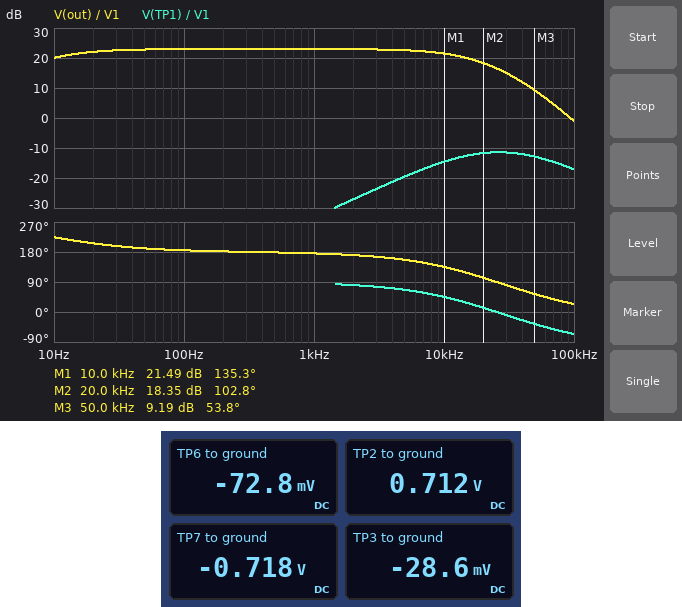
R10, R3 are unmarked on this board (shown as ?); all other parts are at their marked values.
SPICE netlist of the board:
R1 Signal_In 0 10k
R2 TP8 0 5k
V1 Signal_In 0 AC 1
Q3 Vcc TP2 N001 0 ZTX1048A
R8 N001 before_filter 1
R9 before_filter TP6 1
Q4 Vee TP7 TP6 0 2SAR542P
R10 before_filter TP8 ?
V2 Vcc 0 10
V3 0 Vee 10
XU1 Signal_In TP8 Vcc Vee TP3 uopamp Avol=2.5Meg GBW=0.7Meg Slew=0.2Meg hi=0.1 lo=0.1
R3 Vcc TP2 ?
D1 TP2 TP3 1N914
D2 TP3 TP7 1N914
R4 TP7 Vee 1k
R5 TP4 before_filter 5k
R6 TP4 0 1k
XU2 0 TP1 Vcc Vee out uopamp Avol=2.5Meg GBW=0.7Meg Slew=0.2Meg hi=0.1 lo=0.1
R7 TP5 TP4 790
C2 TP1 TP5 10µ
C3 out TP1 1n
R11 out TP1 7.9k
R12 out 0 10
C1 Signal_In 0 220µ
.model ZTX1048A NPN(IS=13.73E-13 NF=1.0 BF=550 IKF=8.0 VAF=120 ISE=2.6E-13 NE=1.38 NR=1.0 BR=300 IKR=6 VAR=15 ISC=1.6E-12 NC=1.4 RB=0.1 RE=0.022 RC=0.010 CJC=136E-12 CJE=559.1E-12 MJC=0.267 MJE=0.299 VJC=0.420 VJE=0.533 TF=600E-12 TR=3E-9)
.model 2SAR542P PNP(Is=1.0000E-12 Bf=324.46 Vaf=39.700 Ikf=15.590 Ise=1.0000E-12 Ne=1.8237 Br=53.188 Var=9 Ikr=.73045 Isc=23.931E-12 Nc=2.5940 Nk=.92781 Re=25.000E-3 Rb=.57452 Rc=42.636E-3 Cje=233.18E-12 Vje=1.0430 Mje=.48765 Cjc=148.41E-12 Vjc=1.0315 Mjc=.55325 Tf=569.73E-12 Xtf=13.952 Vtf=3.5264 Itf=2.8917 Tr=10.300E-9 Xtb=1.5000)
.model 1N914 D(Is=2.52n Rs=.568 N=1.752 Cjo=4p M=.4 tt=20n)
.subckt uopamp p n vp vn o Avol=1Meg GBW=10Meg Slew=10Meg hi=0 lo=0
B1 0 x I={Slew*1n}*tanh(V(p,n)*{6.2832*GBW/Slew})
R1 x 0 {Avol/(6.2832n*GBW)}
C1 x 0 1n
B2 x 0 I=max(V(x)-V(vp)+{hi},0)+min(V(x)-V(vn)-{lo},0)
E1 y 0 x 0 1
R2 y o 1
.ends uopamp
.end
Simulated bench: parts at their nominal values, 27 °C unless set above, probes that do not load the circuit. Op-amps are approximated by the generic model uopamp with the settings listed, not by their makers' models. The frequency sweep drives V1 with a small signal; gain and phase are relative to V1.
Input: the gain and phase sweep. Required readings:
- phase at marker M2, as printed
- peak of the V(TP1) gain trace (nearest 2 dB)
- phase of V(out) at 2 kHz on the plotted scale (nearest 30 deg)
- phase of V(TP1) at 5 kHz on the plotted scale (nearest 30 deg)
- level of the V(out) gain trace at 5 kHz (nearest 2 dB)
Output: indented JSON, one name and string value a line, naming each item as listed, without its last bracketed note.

{
  "phase at marker M2, as printed": "102.8 deg",
  "peak of the V(TP1) gain trace": "-12 dB",
  "phase of V(out) at 2 kHz on the plotted scale": "180 deg",
  "phase of V(TP1) at 5 kHz on the plotted scale": "60 deg",
  "level of the V(out) gain trace at 5 kHz": "22 dB"
}
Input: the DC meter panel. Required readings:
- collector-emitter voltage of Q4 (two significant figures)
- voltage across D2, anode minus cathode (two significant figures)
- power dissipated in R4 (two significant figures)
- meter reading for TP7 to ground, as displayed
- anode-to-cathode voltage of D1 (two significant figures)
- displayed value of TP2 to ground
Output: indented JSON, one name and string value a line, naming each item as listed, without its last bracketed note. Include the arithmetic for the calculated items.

{
  "collector-emitter voltage of Q4": "-10 V - (-72.8 mV) = -9.9 V",
  "voltage across D2, anode minus cathode": "-28.6 mV - (-718 mV) = 690 mV",
  "power dissipated in R4": "(-718 mV - (-10 V))^2 / 1 kΩ = 86 mW",
  "meter reading for TP7 to ground, as displayed": "-0.718 V",
  "anode-to-cathode voltage of D1": "712 mV - (-28.6 mV) = 740 mV",
  "displayed value of TP2 to ground": "0.712 V"
}
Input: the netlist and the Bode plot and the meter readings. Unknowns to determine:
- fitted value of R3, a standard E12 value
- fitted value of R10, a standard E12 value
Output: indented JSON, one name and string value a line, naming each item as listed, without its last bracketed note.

{
  "fitted value of R3, a standard E12 value": "390 Ω",
  "fitted value of R10, a standard E12 value": "82 kΩ"
}
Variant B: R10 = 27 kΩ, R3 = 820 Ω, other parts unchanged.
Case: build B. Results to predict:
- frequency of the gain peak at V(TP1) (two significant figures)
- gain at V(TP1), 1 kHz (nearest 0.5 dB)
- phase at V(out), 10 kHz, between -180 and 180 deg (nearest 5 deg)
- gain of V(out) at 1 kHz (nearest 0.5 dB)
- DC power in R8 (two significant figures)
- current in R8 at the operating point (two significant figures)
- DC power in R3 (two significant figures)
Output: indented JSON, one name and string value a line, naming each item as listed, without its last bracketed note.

{
  "frequency of the gain peak at V(TP1)": "43 kHz",
  "gain at V(TP1), 1 kHz": "-42.0 dB",
  "phase at V(out), 10 kHz, between -180 and 180 deg": "145 deg",
  "gain of V(out) at 1 kHz": "14.5 dB",
  "DC power in R8": "3.4 mW",
  "current in R8 at the operating point": "59 mA",
  "DC power in R3": "110 mW"
}
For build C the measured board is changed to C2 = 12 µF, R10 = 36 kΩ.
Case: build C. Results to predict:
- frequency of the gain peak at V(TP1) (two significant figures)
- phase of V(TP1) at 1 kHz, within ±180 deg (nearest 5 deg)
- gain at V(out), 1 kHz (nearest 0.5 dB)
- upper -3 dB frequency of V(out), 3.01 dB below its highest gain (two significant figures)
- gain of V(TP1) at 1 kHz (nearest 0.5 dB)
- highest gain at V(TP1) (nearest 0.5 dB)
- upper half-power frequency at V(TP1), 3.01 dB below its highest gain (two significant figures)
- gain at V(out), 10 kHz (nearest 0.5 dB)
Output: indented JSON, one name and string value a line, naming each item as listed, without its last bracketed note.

{
  "frequency of the gain peak at V(TP1)": "38 kHz",
  "phase of V(TP1) at 1 kHz, within ±180 deg": "85 deg",
  "gain at V(out), 1 kHz": "16.5 dB",
  "upper -3 dB frequency of V(out), 3.01 dB below its highest gain": "17 kHz",
  "gain of V(TP1) at 1 kHz": "-39.5 dB",
  "highest gain at V(TP1)": "-16.5 dB",
  "upper half-power frequency at V(TP1), 3.01 dB below its highest gain": "110 kHz",
  "gain at V(out), 10 kHz": "15.0 dB"
}
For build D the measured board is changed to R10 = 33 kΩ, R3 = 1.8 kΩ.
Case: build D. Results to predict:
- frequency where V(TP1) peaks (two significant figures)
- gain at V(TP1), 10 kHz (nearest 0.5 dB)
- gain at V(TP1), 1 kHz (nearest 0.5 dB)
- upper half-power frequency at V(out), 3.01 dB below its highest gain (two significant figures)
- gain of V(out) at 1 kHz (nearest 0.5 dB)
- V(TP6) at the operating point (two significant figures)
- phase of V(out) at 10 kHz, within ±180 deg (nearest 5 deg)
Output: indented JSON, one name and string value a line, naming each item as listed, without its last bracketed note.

{
  "frequency where V(TP1) peaks": "40 kHz",
  "gain at V(TP1), 10 kHz": "-21.5 dB",
  "gain at V(TP1), 1 kHz": "-40.5 dB",
  "upper half-power frequency at V(out), 3.01 dB below its highest gain": "17 kHz",
  "gain of V(out) at 1 kHz": "16.0 dB",
  "V(TP6) at the operating point": "-46 mV",
  "phase of V(out) at 10 kHz, within ±180 deg": "145 deg"
}
